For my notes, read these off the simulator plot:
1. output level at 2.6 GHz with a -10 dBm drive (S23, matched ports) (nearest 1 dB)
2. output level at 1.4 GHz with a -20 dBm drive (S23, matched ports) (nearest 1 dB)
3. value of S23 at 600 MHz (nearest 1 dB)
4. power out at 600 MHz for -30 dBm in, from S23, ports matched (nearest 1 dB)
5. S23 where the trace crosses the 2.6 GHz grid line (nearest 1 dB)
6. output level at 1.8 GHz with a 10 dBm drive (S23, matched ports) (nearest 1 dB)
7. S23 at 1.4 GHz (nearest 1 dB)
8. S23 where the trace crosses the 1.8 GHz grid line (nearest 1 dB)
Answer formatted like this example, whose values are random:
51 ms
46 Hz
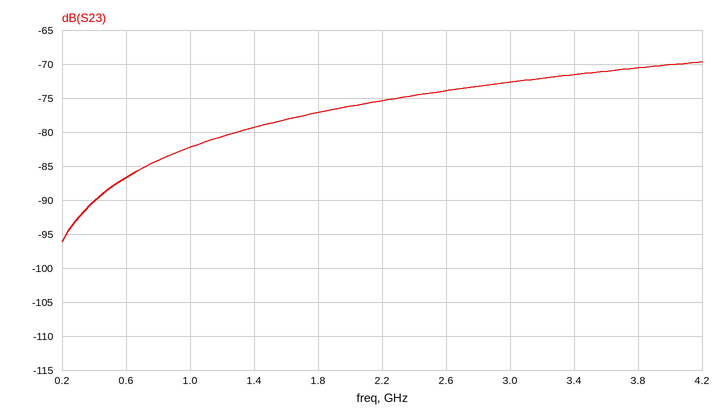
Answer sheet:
-84 dBm
-99 dBm
-87 dB
-117 dBm
-74 dB
-67 dBm
-79 dB
-77 dB
